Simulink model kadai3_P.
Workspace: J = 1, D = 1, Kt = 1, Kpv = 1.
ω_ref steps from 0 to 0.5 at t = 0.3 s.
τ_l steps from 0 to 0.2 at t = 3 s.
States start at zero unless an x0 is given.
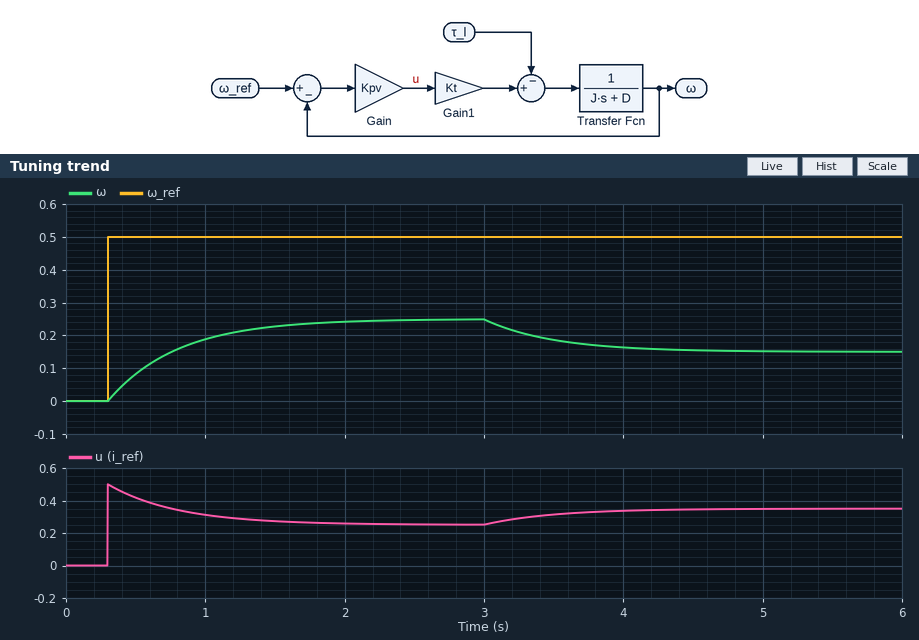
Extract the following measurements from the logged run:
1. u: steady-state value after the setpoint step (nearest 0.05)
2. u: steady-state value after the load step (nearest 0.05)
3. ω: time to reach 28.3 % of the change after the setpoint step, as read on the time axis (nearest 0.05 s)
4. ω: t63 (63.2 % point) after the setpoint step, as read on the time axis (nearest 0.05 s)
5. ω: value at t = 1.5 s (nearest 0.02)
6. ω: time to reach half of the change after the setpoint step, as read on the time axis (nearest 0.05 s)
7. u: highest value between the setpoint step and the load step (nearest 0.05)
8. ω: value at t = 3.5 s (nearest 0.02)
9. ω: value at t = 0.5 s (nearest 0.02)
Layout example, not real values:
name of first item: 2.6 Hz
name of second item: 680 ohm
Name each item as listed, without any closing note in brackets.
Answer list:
u: steady-state value after the setpoint step: 0.25
u: steady-state value after the load step: 0.35
ω: time to reach 28.3 % of the change after the setpoint step, as read on the time axis: 0.45 s
ω: t63 (63.2 % point) after the setpoint step, as read on the time axis: 0.80 s
ω: value at t = 1.5 s: 0.22
ω: time to reach half of the change after the setpoint step, as read on the time axis: 0.65 s
u: highest value between the setpoint step and the load step: 0.50
ω: value at t = 3.5 s: 0.18
ω: value at t = 0.5 s: 0.08
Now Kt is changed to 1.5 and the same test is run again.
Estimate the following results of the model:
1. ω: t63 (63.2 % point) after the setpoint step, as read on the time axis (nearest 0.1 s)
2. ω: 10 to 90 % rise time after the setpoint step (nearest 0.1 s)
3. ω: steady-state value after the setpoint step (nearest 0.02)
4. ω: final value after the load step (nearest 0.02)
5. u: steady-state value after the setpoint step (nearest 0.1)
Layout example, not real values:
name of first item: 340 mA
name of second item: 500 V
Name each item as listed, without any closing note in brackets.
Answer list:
ω: t63 (63.2 % point) after the setpoint step, as read on the time axis: 0.7 s
ω: 10 to 90 % rise time after the setpoint step: 0.9 s
ω: steady-state value after the setpoint step: 0.30
ω: final value after the load step: 0.22
u: steady-state value after the setpoint step: 0.2
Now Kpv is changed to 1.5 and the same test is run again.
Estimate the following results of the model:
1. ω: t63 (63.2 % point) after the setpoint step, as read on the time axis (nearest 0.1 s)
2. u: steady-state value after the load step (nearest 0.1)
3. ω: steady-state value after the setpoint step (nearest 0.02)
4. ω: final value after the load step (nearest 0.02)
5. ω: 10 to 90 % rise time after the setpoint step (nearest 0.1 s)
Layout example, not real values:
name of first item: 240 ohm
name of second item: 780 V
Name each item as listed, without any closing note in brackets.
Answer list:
ω: t63 (63.2 % point) after the setpoint step, as read on the time axis: 0.7 s
u: steady-state value after the load step: 0.4
ω: steady-state value after the setpoint step: 0.30
ω: final value after the load step: 0.22
ω: 10 to 90 % rise time after the setpoint step: 0.9 s
